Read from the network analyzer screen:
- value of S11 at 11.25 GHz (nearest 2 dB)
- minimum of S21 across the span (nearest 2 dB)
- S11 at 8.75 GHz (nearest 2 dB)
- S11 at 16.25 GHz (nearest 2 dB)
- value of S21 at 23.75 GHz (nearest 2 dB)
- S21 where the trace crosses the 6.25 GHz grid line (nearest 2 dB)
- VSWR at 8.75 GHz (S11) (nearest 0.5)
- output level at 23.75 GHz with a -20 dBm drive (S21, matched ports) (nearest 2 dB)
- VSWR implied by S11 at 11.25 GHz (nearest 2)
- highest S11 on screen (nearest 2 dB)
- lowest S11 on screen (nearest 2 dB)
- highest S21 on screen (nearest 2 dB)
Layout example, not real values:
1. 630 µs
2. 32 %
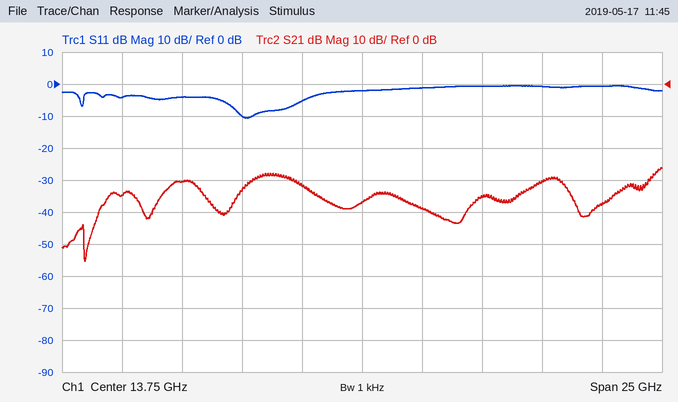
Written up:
1. -6 dB
2. -56 dB
3. -10 dB
4. -2 dB
5. -38 dB
6. -30 dB
7. 2.0
8. -58 dBm
9. 4
10. 0 dB
11. -10 dB
12. -26 dB
